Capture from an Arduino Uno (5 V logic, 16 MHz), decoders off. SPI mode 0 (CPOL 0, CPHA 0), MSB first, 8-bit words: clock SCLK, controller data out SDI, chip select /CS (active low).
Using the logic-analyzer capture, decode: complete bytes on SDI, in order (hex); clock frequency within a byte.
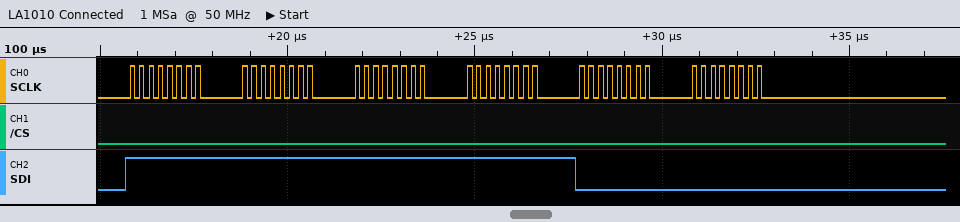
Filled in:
0xFF 0xFF 0xFF 0xFF 0x00 0x00
4 MHz
